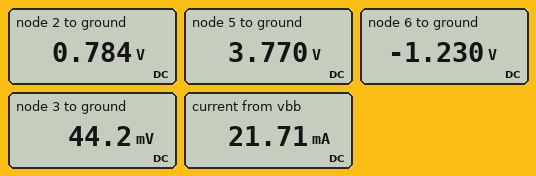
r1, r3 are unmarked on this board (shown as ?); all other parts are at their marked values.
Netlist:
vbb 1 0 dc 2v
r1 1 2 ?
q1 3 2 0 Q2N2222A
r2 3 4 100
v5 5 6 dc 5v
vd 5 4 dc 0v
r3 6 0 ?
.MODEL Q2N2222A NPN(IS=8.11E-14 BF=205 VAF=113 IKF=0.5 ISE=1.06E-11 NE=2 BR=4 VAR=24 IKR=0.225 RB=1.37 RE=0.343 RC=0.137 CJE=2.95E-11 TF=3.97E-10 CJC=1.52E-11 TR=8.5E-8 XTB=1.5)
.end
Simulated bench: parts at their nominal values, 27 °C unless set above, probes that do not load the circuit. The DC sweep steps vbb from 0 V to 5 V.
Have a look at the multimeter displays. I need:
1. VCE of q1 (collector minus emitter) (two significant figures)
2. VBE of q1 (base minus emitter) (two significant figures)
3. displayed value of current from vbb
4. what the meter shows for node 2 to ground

44 mV
780 mV
21.71 mA
0.784 V
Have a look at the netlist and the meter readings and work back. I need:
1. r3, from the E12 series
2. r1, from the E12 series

33 Ω
56 Ω
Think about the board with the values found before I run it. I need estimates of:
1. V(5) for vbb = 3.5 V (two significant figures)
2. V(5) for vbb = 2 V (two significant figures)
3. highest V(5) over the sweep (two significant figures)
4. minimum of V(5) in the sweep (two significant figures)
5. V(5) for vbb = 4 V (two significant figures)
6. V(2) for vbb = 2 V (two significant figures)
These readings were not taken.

3.8 V
3.8 V
5.0 V
3.8 V
3.8 V
780 mV
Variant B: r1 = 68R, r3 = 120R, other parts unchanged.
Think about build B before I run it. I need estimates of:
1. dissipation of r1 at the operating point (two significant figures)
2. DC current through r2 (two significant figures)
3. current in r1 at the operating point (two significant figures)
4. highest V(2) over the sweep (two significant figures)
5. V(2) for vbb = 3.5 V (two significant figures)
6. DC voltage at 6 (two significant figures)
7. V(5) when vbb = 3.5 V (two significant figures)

22 mW
23 mA
18 mA
870 mV
820 mV
-2.7 V
2.3 V
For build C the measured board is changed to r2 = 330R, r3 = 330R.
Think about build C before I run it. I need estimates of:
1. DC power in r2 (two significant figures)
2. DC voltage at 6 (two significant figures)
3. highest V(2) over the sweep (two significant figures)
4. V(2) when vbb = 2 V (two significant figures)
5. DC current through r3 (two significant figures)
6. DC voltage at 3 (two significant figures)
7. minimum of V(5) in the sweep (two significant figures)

19 mW
-2.5 V
890 mV
770 mV
7.5 mA
22 mV
2.5 V
